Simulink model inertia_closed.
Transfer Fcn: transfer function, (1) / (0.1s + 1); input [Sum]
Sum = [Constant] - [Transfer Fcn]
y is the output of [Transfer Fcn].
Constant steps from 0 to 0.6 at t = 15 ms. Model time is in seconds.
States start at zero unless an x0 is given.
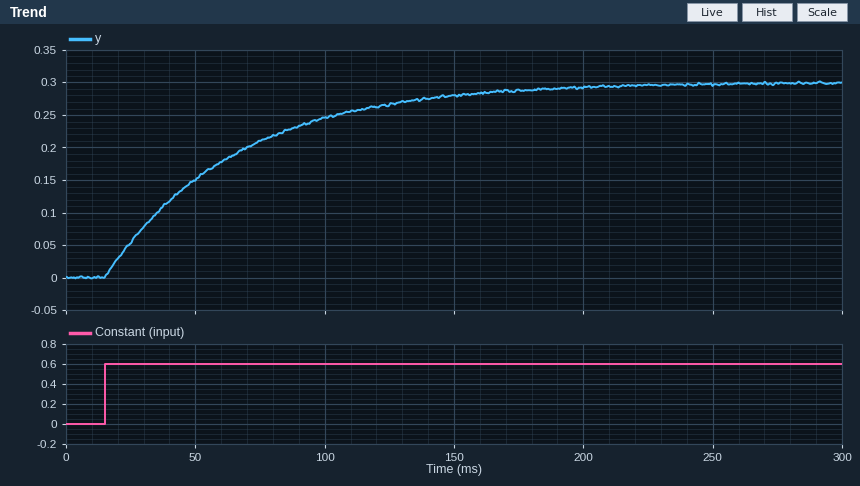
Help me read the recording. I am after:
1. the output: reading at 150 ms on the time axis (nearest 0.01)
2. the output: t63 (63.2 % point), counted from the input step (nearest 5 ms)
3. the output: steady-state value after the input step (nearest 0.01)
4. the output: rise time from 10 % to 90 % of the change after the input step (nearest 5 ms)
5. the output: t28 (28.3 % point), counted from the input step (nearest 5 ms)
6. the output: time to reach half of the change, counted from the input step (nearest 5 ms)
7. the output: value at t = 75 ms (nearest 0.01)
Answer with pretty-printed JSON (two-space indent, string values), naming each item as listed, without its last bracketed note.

{
  "the output: reading at 150 ms on the time axis": "0.28",
  "the output: t63 (63.2 % point), counted from the input step": "50 ms",
  "the output: steady-state value after the input step": "0.30",
  "the output: rise time from 10 % to 90 % of the change after the input step": "110 ms",
  "the output: t28 (28.3 % point), counted from the input step": "15 ms",
  "the output: time to reach half of the change, counted from the input step": "35 ms",
  "the output: value at t = 75 ms": "0.21"
}
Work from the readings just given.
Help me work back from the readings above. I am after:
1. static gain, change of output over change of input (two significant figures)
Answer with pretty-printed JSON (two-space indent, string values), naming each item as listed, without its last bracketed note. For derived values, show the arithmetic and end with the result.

{
  "static gain, change of output over change of input": "(0.3 - 0) / (0.6 - 0) = 0.50"
}
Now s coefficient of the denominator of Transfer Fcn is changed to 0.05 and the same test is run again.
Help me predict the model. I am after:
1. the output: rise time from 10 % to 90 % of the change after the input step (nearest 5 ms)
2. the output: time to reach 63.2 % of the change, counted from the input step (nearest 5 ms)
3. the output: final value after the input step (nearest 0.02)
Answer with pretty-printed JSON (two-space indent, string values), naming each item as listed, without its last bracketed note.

{
  "the output: rise time from 10 % to 90 % of the change after the input step": "55 ms",
  "the output: time to reach 63.2 % of the change, counted from the input step": "25 ms",
  "the output: final value after the input step": "0.30"
}
